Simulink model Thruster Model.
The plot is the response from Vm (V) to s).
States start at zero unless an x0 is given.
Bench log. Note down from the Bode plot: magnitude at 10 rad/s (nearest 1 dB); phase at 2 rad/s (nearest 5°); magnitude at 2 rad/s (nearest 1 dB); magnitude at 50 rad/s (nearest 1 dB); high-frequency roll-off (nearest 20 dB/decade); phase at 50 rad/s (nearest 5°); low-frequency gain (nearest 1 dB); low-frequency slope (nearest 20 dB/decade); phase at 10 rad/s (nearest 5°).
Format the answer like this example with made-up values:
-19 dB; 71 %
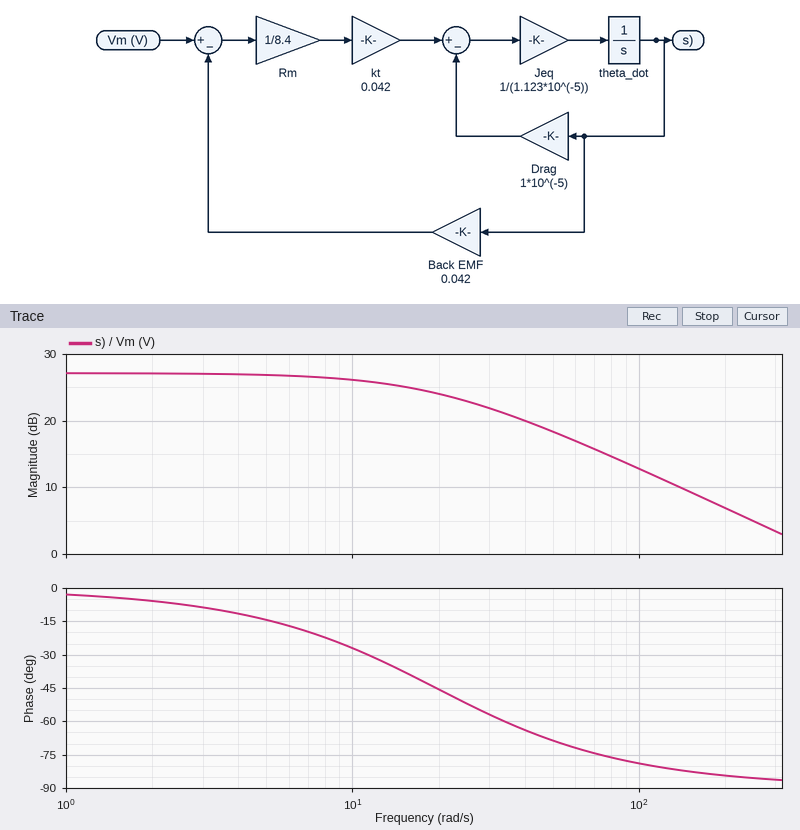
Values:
26 dB; -5°; 27 dB; 18 dB; -20 dB/decade; -70°; 27 dB; 0 dB/decade; -25°
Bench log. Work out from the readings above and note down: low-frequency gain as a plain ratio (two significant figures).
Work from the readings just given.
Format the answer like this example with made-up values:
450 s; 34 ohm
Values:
22
